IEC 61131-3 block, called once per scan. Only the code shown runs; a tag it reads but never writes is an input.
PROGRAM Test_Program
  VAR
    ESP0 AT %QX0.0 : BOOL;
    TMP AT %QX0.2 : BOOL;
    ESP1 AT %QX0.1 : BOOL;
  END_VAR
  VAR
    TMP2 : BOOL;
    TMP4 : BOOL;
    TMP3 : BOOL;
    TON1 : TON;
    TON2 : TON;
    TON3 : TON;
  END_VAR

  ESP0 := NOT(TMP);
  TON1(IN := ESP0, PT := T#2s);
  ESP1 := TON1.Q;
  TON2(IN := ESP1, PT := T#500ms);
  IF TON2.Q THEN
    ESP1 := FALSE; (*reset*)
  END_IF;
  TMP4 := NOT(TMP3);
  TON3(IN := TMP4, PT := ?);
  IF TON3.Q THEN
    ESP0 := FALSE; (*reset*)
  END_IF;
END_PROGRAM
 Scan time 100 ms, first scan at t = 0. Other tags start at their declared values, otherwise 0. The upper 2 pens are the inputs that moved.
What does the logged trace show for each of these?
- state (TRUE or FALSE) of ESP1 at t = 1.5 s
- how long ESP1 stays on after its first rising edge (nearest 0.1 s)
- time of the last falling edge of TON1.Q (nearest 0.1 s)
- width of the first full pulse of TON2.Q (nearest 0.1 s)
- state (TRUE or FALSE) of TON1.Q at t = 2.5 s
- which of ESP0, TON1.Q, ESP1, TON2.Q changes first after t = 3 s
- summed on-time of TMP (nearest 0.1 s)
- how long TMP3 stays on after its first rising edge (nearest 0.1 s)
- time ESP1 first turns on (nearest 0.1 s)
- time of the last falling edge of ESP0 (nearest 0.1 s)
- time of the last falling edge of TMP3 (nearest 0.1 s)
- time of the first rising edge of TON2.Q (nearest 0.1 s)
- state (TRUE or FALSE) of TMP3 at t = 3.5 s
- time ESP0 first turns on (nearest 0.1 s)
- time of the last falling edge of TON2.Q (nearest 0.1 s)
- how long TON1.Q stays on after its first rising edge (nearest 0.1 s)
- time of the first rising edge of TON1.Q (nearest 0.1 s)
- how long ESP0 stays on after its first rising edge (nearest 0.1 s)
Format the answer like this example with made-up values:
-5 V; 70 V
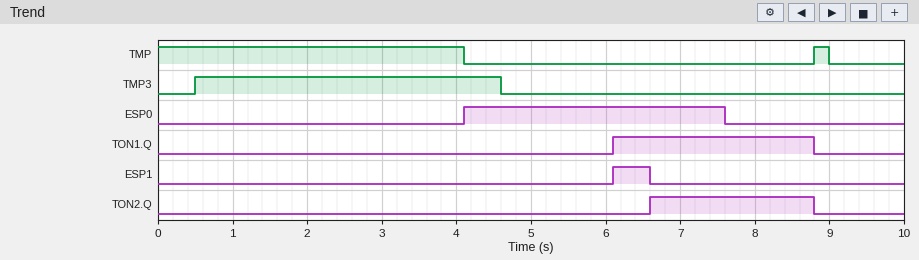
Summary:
FALSE; 0.5 s; 8.8 s; 2.2 s; FALSE; ESP0; 4.3 s; 4.1 s; 6.1 s; 7.6 s; 4.6 s; 6.6 s; TRUE; 4.1 s; 8.8 s; 2.7 s; 6.1 s; 3.5 s
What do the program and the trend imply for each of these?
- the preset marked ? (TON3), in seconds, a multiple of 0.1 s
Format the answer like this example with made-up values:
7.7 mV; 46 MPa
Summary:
3.0 s
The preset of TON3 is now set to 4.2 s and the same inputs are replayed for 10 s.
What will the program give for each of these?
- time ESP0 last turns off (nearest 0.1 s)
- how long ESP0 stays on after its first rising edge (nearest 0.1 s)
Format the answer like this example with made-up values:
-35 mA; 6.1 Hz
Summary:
8.8 s; 4.7 s
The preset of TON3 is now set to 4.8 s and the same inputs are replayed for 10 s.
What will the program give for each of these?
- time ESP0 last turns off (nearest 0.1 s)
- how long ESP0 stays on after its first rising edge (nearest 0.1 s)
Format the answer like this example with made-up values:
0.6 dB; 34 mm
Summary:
9.4 s; 4.7 s
